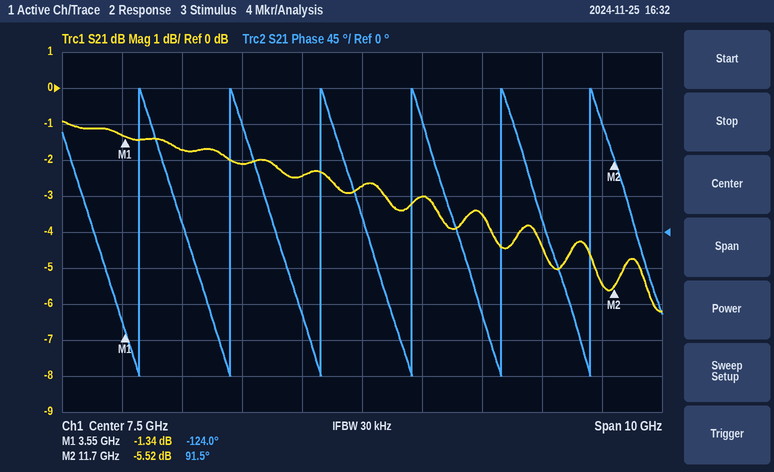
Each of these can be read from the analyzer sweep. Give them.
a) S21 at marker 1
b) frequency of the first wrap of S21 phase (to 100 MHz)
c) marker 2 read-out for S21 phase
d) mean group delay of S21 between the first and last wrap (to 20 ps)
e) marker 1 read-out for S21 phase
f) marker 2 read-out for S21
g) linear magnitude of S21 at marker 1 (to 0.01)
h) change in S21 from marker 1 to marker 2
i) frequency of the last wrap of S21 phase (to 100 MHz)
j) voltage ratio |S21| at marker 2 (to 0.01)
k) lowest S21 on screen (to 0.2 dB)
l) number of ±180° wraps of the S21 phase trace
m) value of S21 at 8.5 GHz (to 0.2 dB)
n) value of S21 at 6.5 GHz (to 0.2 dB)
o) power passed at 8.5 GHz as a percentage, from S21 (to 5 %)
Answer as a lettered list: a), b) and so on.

a) -1.34 dB
b) 3.8 GHz
c) 91.5°
d) 660 ps
e) -124.0°
f) -5.52 dB
g) 0.86
h) -4.18 dB
i) 11.3 GHz
j) 0.53
k) -6.2 dB
l) 6
m) -3.0 dB
n) -2.4 dB
o) 50 %
